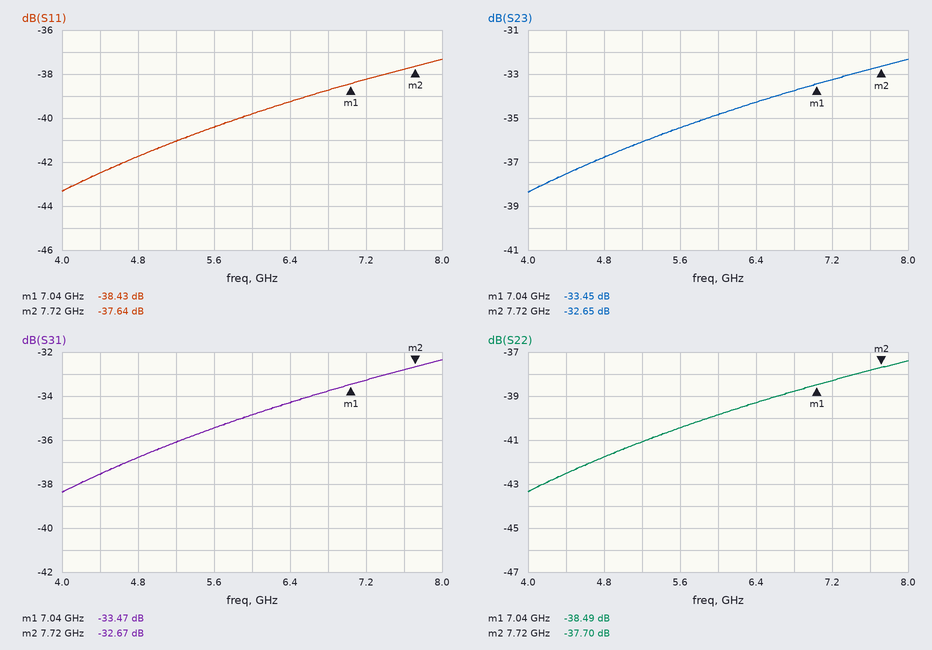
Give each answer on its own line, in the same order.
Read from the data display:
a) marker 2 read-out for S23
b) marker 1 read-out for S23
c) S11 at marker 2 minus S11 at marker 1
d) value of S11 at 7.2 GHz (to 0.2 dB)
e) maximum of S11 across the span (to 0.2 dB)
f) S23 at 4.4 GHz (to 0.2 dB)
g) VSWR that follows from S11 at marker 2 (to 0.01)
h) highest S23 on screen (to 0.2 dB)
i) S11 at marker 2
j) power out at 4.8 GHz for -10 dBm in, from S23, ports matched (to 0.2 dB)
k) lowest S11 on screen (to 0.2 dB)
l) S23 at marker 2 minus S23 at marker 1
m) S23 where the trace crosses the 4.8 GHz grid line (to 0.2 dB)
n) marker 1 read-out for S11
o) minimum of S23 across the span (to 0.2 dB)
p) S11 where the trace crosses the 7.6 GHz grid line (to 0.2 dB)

-32.65 dB
-33.45 dB
0.79 dB
-38.2 dB
-37.4 dB
-37.6 dB
1.03
-32.4 dB
-37.64 dB
-46.8 dBm
-43.4 dB
0.80 dB
-36.8 dB
-38.43 dB
-38.4 dB
-37.8 dB
